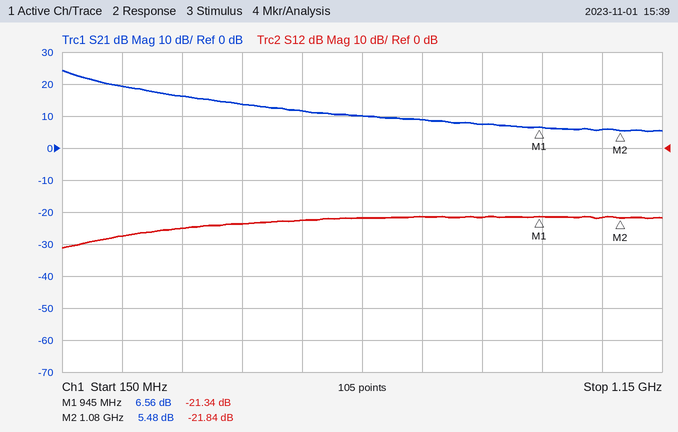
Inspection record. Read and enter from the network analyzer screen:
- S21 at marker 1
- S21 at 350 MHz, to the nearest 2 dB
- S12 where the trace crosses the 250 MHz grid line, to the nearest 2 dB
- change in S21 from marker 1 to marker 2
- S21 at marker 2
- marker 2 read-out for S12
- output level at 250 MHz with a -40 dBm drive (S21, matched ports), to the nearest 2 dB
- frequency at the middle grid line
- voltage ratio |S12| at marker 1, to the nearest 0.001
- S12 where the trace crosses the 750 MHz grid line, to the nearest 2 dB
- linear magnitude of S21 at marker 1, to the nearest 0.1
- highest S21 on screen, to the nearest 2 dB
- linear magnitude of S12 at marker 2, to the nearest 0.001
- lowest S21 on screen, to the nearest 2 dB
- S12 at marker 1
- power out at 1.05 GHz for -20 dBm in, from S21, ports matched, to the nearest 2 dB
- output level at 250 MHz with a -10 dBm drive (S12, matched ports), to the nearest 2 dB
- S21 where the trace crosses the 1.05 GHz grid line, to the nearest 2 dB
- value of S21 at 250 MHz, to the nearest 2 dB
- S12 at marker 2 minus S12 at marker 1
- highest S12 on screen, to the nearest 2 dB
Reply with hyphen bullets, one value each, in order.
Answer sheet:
- 6.56 dB
- 16 dB
- -28 dB
- -1.08 dB
- 5.48 dB
- -21.84 dB
- -20 dBm
- 650 MHz
- 0.086
- -22 dB
- 2.1
- 24 dB
- 0.081
- 6 dB
- -21.34 dB
- -14 dBm
- -38 dBm
- 6 dB
- 20 dB
- -0.50 dB
- -22 dB
